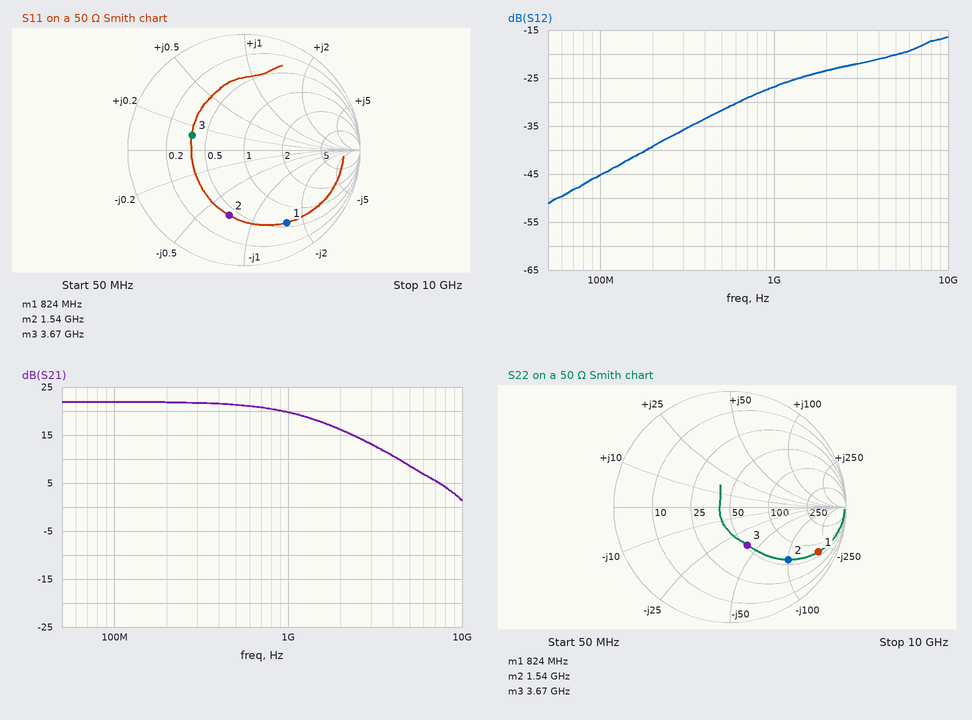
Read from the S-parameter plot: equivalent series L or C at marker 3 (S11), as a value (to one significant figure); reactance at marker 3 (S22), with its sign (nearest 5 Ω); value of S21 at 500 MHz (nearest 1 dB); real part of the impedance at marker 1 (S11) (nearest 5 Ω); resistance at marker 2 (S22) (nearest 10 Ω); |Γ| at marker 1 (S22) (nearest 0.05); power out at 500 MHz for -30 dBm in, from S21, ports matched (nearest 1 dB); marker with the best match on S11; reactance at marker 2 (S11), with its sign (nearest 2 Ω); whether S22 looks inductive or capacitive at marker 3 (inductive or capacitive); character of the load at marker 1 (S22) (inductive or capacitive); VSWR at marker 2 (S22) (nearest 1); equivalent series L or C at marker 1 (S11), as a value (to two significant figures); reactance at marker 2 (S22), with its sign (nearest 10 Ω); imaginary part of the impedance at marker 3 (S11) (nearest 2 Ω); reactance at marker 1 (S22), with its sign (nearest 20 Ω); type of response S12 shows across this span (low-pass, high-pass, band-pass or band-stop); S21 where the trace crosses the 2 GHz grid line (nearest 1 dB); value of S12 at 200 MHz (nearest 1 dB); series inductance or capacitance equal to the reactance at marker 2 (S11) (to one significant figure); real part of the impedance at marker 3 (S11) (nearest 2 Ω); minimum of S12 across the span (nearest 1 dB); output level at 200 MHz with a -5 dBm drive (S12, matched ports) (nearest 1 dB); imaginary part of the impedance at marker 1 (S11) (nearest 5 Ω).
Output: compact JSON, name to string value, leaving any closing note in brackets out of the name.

{"equivalent series L or C at marker 3 (S11), as a value": "300 pH", "reactance at marker 3 (S22), with its sign": "-40 Ω", "value of S21 at 500 MHz": "21 dB", "real part of the impedance at marker 1 (S11)": "30 Ω", "resistance at marker 2 (S22)": "60 Ω", "|Γ| at marker 1 (S22)": "0.85", "power out at 500 MHz for -30 dBm in, from S21, ports matched": "-9 dBm", "marker with the best match on S11": "marker 3", "reactance at marker 2 (S11), with its sign": "-36 Ω", "whether S22 looks inductive or capacitive at marker 3": "capacitive", "character of the load at marker 1 (S22)": "capacitive", "VSWR at marker 2 (S22)": "5", "equivalent series L or C at marker 1 (S11), as a value": "2.4 pF", "reactance at marker 2 (S22), with its sign": "-100 Ω", "imaginary part of the impedance at marker 3 (S11)": "+6 Ω", "reactance at marker 1 (S22), with its sign": "-180 Ω", "type of response S12 shows across this span": "high-pass", "S21 where the trace crosses the 2 GHz grid line": "16 dB", "value of S12 at 200 MHz": "-39 dB", "series inductance or capacitance equal to the reactance at marker 2 (S11)": "3 pF", "real part of the impedance at marker 3 (S11)": "18 Ω", "minimum of S12 across the span": "-51 dB", "output level at 200 MHz with a -5 dBm drive (S12, matched ports)": "-44 dBm", "imaginary part of the impedance at marker 1 (S11)": "-80 Ω"}
